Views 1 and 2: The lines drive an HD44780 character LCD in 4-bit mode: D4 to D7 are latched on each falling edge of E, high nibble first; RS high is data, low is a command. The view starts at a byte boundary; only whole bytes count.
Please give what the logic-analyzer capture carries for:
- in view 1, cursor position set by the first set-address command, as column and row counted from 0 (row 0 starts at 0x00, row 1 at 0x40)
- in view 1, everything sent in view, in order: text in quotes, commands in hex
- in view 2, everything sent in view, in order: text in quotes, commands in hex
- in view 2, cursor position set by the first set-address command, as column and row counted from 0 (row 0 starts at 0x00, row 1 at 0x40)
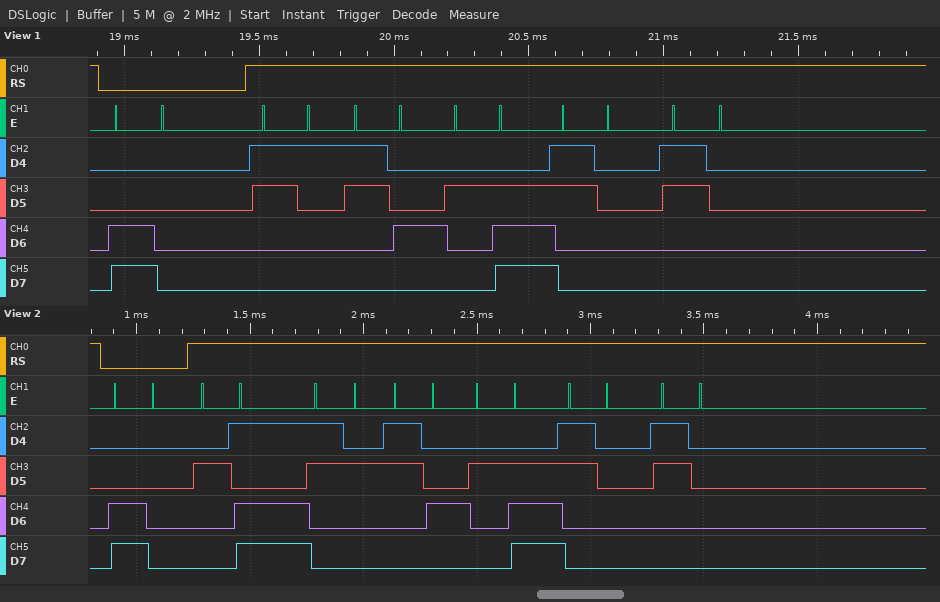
column 0, row 1
0xC0 "14.00"
0xC0 "-24.00"
column 0, row 1
